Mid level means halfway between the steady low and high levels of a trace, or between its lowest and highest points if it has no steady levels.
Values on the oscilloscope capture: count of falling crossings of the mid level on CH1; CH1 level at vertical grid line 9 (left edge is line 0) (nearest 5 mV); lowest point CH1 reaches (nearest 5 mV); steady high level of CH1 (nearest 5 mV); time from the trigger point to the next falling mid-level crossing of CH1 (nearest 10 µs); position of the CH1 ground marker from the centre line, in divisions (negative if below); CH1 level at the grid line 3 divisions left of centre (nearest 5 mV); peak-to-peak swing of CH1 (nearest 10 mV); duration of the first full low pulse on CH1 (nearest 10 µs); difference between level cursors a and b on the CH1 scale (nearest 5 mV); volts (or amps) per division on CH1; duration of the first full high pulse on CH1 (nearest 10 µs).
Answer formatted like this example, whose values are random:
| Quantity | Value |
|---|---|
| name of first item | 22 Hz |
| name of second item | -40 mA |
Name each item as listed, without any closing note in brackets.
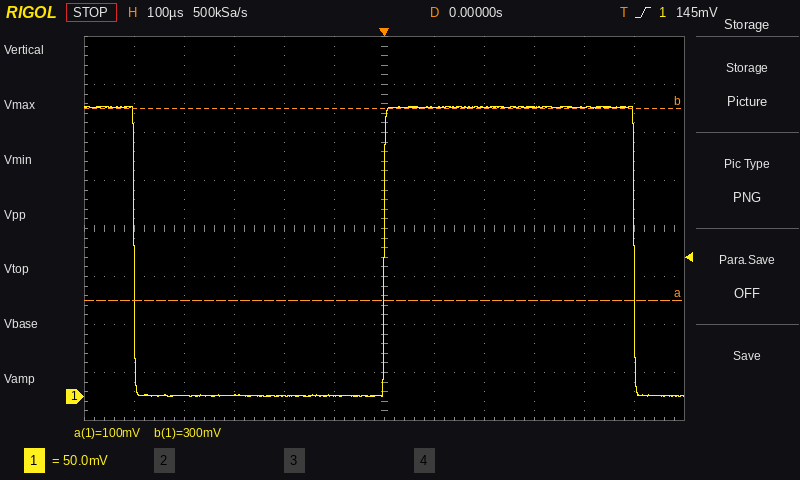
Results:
| Quantity | Value |
|---|---|
| count of falling crossings of the mid level on CH1 | 2 |
| CH1 level at vertical grid line 9 (left edge is line 0) | 300 mV |
| lowest point CH1 reaches | 0 mV |
| steady high level of CH1 | 300 mV |
| time from the trigger point to the next falling mid-level crossing of CH1 | 500 µs |
| position of the CH1 ground marker from the centre line, in divisions | -3.5 div |
| CH1 level at the grid line 3 divisions left of centre | 0 mV |
| peak-to-peak swing of CH1 | 300 mV |
| duration of the first full low pulse on CH1 | 500 µs |
| difference between level cursors a and b on the CH1 scale | 200 mV |
| volts (or amps) per division on CH1 | 50 mV |
| duration of the first full high pulse on CH1 | 500 µs |
